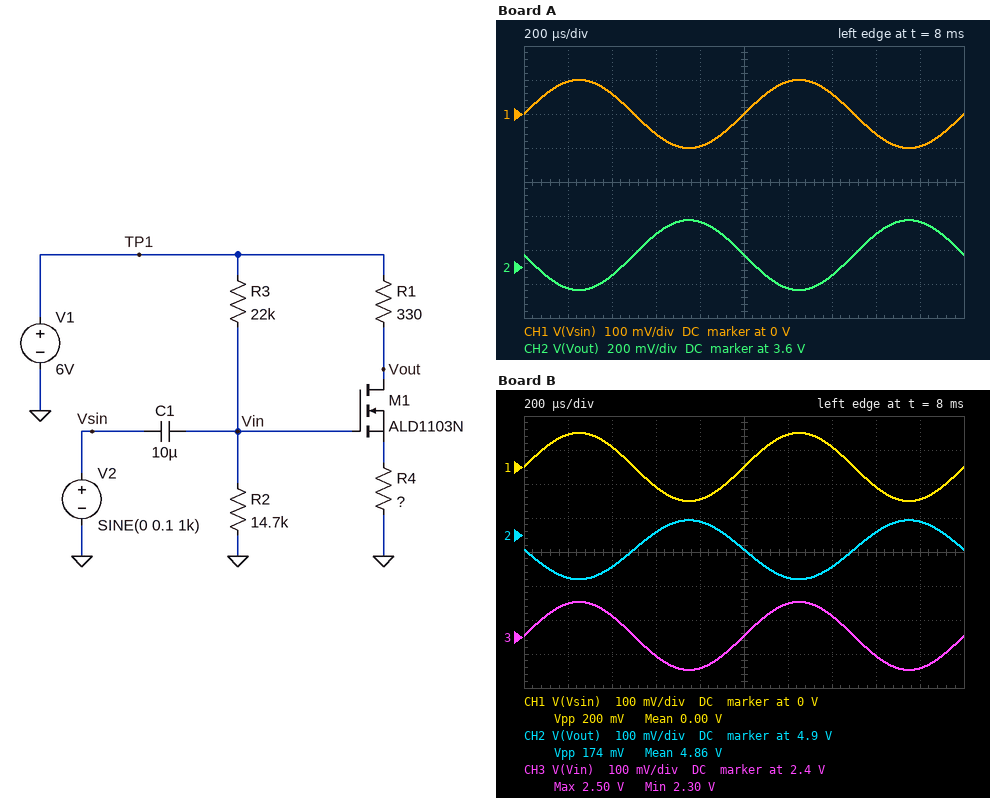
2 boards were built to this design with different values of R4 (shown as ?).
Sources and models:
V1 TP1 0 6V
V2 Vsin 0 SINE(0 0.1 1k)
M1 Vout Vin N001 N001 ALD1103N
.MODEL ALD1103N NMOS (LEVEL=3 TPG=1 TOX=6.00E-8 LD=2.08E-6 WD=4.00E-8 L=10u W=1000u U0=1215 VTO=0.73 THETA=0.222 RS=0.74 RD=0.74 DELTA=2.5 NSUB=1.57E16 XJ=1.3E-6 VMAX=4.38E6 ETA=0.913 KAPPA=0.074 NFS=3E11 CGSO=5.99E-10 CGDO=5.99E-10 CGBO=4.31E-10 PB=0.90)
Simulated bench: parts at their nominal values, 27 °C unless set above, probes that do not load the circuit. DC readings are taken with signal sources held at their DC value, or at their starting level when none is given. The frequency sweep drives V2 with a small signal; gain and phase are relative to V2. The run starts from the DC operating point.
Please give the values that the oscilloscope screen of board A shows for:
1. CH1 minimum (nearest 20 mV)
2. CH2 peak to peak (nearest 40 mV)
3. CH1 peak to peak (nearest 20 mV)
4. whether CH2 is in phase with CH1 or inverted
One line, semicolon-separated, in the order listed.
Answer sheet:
-100 mV; 400 mV; 200 mV; inverted
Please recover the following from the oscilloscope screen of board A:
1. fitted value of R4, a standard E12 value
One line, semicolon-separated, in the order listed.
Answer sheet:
39 Ω
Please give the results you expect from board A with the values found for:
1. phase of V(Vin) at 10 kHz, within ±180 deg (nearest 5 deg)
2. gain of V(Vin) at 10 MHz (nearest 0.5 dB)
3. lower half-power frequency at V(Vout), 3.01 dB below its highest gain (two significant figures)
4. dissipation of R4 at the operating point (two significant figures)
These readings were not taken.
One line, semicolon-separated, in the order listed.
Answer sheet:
0 deg; 0 dB; 1.8 Hz; 1.9 mW
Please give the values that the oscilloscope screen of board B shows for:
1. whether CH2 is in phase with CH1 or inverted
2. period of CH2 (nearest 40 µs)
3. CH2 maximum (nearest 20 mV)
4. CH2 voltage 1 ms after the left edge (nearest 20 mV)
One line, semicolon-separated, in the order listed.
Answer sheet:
inverted; 1.00 ms; 4.94 V; 4.86 V
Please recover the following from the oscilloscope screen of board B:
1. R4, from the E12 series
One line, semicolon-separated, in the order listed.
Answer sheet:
220 Ω
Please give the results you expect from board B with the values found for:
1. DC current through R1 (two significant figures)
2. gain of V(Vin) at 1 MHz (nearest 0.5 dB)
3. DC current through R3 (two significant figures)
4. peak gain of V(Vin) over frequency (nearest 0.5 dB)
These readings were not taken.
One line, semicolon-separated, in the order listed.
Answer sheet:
3.5 mA; 0 dB; 160 µA; 0 dB
